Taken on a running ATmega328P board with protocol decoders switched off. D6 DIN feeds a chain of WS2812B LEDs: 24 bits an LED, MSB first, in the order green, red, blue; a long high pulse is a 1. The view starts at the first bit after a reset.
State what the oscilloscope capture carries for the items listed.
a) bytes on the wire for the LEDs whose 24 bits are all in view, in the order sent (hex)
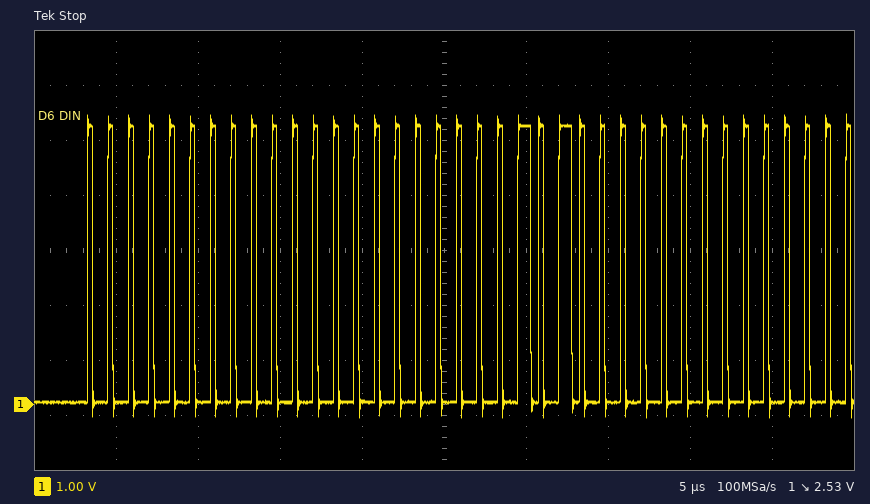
00 00 05
